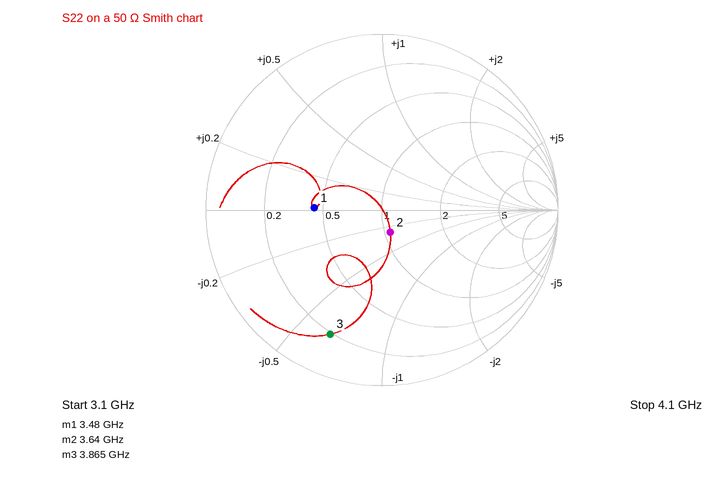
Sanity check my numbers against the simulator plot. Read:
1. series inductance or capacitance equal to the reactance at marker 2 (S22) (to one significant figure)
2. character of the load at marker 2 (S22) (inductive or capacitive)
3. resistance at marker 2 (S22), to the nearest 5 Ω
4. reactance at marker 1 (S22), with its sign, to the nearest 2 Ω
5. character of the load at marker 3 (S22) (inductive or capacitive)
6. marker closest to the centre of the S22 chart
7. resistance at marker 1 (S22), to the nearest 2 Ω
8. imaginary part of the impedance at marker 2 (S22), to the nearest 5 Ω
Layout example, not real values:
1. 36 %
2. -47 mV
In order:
1. 3 pF
2. capacitive
3. 55 Ω
4. 0 Ω
5. capacitive
6. marker 2
7. 22 Ω
8. -15 Ω
